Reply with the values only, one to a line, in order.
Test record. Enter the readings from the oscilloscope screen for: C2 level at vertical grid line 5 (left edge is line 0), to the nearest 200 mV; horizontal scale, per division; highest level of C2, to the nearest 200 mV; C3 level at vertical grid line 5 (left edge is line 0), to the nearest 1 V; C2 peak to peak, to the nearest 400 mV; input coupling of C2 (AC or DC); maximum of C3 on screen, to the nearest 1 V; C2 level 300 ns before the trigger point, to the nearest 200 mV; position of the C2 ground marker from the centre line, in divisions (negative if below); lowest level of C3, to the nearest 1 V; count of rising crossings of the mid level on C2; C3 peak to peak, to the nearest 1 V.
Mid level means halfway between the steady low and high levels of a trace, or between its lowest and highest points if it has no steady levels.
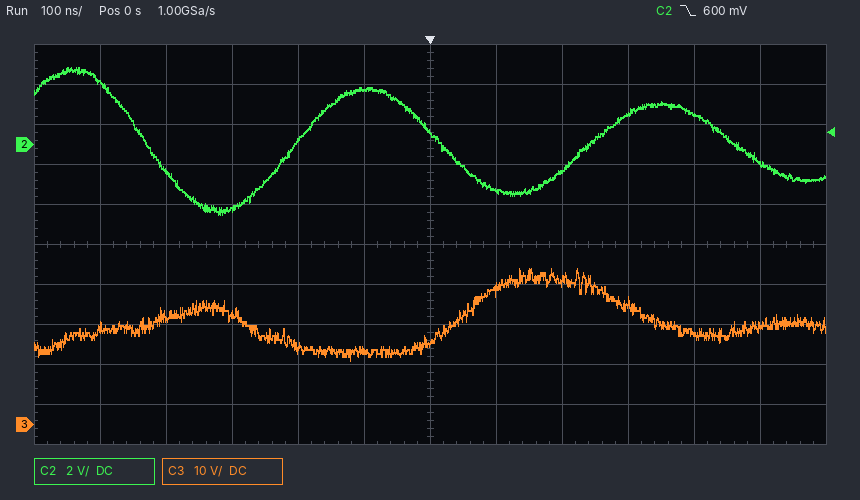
2.8 V
100 ns
3.8 V
19 V
7.2 V
DC
39 V
-3.2 V
+2.5 div
16 V
2
23 V
